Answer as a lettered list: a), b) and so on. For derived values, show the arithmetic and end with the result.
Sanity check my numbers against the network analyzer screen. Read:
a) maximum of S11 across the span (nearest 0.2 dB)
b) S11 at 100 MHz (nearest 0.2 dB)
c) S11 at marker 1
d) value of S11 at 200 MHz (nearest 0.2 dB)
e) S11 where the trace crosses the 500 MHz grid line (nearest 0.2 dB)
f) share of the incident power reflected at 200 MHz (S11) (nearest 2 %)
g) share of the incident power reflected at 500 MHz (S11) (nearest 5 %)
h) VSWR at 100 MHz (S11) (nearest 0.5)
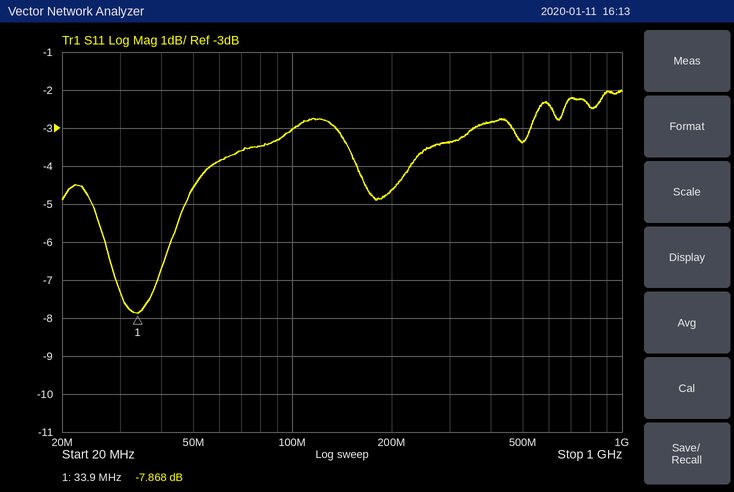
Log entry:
a) -2.0 dB
b) -3.0 dB
c) -7.868 dB
d) -4.6 dB
e) -3.4 dB
f) 10^(-4.6/10) ≈ 34.7 %, so 34 % to the nearest 2 %
g) 10^(-3.4/10) ≈ 45.7 %, so 45 % to the nearest 5 %
h) |Γ| = 10^(-3/20) = 0.7079; VSWR = (1 + 0.7079)/(1 − 0.7079) ≈ 5.85, so 6.0 to the nearest 0.5
